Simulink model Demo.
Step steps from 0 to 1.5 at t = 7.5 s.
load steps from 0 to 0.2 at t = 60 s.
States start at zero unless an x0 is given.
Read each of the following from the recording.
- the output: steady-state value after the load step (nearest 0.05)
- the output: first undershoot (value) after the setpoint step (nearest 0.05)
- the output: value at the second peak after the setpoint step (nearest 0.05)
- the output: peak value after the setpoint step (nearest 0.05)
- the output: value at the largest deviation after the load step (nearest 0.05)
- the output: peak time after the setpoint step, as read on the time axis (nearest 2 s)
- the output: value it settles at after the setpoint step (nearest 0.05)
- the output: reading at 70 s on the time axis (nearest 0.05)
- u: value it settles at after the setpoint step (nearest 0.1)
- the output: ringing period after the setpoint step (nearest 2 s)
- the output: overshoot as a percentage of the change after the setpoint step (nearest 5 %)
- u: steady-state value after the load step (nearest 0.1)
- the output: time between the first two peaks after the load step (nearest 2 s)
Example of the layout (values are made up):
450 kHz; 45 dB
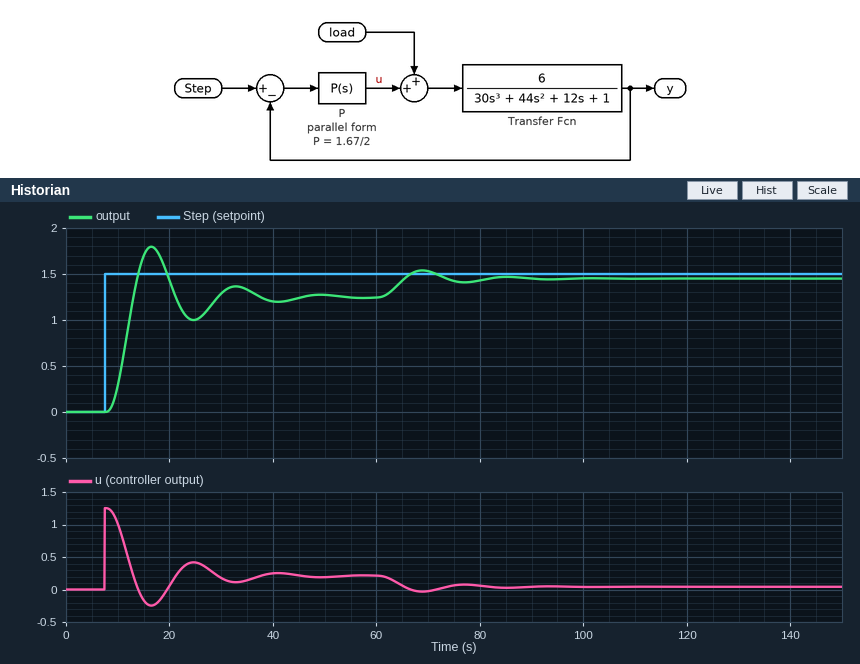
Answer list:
1.45; 1.00; 1.35; 1.80; 1.55; 16 s; 1.25; 1.55; 0.2; 16 s; 45 %; 0.0; 16 s
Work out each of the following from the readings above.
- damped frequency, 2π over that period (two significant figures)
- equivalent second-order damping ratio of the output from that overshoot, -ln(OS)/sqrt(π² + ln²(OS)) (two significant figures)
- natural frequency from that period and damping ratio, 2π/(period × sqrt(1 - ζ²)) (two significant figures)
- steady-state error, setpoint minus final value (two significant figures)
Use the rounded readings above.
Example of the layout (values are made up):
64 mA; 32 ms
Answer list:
0.39 rad/s; 0.25; 0.41 rad/s; 0.25
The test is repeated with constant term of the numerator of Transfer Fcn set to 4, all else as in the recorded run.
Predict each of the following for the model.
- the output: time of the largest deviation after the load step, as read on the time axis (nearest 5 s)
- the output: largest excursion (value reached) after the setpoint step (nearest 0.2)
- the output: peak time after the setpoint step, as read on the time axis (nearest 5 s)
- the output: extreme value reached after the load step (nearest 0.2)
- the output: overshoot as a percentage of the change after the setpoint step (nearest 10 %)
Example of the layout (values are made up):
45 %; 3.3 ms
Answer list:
70 s; 1.6; 20 s; 1.4; 30 %
